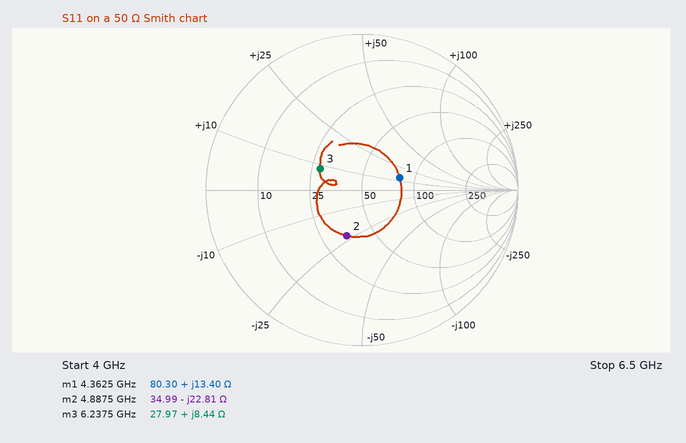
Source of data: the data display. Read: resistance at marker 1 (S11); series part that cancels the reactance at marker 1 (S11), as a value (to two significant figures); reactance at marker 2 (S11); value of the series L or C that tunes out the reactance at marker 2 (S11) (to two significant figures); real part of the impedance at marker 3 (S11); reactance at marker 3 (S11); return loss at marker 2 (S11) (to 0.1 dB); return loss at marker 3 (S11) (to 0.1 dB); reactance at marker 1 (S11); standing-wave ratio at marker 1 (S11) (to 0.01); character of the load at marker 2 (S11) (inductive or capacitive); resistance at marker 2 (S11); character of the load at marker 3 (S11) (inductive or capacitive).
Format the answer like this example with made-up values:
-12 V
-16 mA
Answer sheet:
80.30 Ω
2.7 pF
-22.81 Ω
740 pH
27.97 Ω
+8.44 Ω
10.2 dB
10.4 dB
+13.40 Ω
1.68
capacitive
34.99 Ω
inductive
